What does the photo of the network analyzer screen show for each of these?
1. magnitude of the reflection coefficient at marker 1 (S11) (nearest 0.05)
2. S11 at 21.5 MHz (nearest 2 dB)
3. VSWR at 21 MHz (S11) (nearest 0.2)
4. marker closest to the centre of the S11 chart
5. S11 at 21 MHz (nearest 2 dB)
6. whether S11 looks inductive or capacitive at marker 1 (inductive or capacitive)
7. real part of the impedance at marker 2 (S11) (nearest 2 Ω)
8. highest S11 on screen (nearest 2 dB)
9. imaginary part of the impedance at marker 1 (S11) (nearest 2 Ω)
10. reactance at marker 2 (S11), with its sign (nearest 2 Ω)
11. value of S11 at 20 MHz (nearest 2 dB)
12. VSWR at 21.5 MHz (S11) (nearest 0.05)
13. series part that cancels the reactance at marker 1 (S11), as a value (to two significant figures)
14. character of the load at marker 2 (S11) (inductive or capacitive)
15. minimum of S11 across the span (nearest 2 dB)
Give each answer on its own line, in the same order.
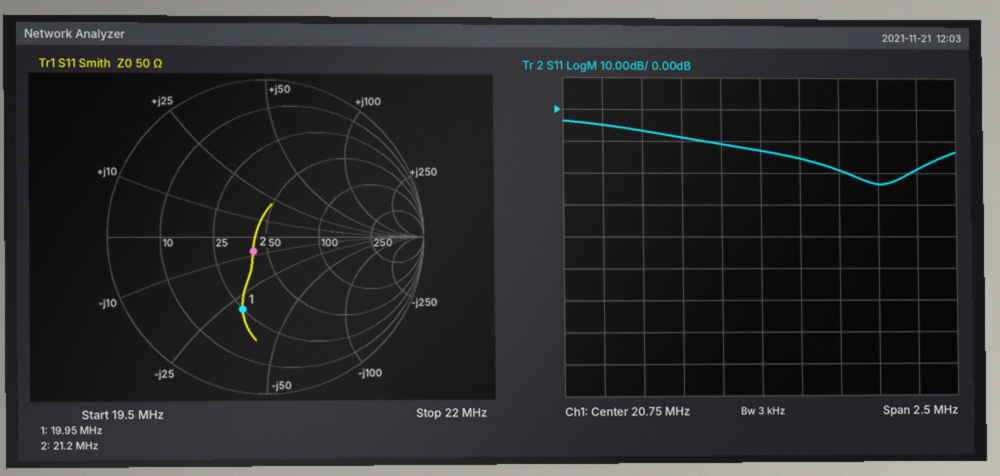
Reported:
0.50
-24 dB
1.4
marker 2
-16 dB
capacitive
42 Ω
-4 dB
-30 Ω
-8 Ω
-6 dB
1.15
240 nH
capacitive
-24 dB
